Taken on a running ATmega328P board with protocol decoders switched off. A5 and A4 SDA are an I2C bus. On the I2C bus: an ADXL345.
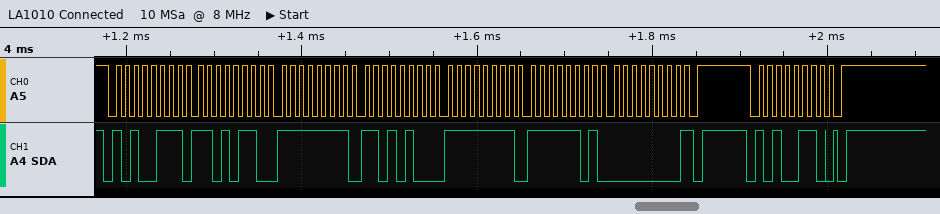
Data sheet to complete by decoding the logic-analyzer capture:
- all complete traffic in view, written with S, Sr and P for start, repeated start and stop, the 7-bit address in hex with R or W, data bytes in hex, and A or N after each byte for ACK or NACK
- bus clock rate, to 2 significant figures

S 53R A D6 A FF A D4 A FF A FD A 00 N P S 53W A P
100 kHz
